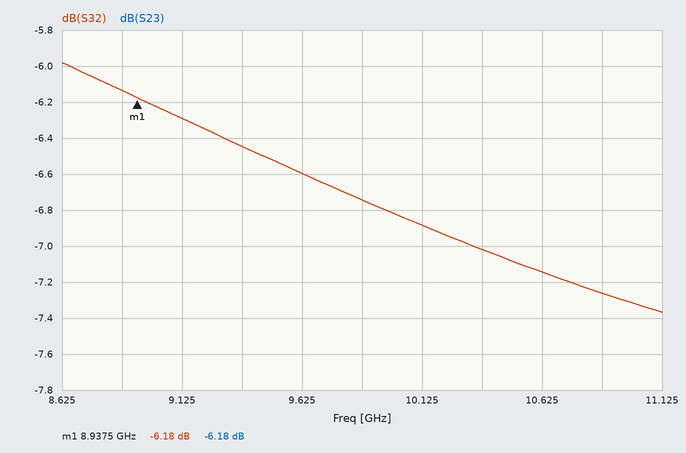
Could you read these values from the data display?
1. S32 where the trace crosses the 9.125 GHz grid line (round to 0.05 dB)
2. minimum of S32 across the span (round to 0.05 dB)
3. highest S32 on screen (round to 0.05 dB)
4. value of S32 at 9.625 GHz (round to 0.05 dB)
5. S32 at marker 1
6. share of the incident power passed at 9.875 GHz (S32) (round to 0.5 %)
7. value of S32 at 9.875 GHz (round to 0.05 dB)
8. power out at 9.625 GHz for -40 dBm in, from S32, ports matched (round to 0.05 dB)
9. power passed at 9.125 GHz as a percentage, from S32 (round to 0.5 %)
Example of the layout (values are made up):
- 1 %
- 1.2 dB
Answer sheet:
- -6.30 dB
- -7.35 dB
- -6.00 dB
- -6.60 dB
- -6.18 dB
- 21.0 %
- -6.75 dB
- -46.60 dBm
- 23.5 %
